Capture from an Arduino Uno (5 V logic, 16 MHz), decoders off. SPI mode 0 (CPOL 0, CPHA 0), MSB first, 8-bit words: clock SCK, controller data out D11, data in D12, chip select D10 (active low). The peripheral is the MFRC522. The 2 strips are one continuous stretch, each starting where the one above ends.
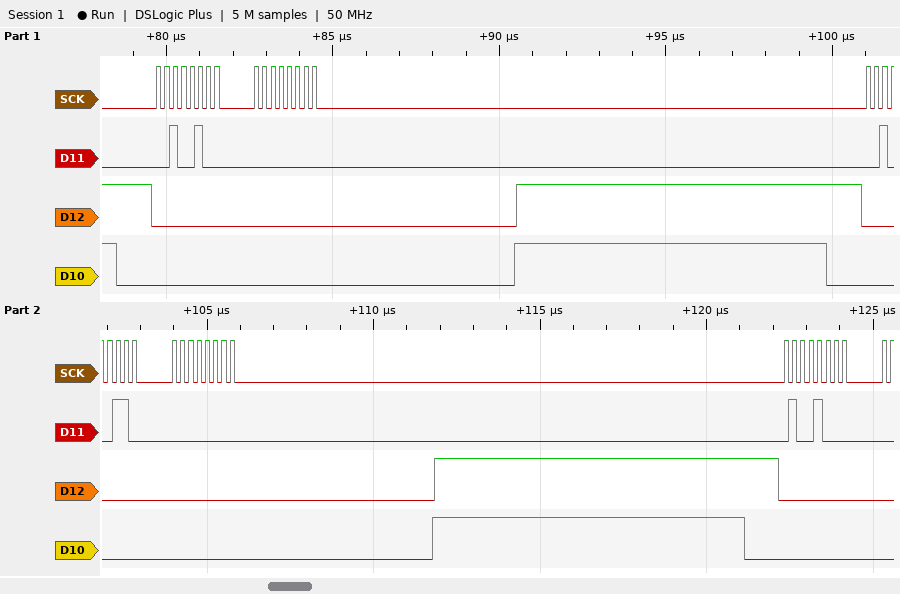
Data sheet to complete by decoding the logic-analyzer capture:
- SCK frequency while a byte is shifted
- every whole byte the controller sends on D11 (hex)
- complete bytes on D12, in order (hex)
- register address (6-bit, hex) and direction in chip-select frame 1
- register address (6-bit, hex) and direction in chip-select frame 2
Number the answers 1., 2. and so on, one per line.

1. 4 MHz
2. 0x24 0x00 0x26 0x00 0x48
3. 0x00 0x00 0x00 0x00 0x00
4. 0x12 write
5. 0x13 write
